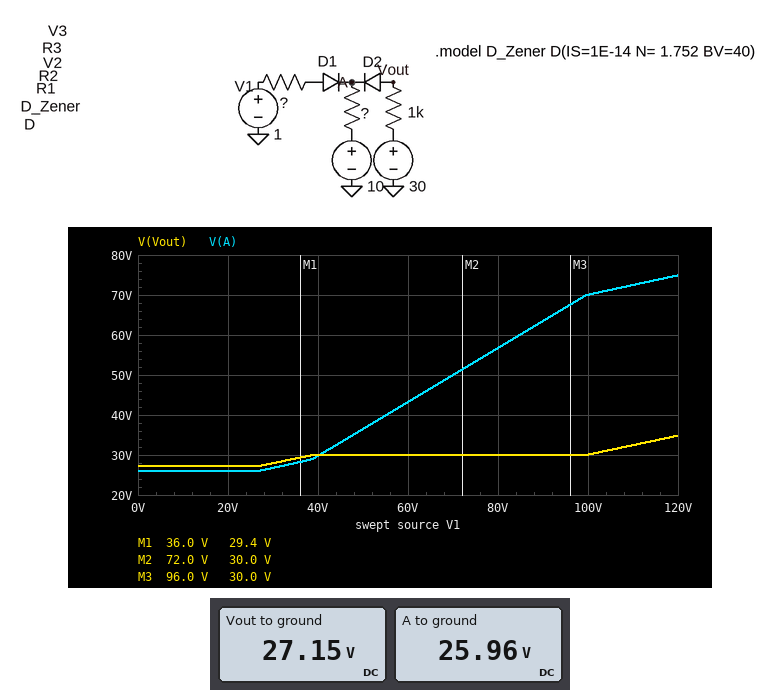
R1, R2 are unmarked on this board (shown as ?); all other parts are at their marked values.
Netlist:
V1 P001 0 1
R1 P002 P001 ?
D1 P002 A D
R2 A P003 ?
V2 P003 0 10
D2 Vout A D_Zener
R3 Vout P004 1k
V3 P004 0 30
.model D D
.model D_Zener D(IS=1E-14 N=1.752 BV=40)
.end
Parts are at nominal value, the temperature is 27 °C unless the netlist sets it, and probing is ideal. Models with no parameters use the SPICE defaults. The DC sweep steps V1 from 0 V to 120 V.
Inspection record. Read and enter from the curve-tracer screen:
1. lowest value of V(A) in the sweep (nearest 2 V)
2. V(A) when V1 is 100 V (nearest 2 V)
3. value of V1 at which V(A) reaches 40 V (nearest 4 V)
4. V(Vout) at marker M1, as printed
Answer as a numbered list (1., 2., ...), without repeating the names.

1. 26 V
2. 70 V
3. 56 V
4. 29.4 V
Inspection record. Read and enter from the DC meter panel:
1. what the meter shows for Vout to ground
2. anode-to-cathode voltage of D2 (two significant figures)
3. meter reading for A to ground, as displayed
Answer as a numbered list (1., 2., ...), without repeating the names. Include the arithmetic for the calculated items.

1. 27.15 V
2. 27.15 V - 25.96 V = 1.2 V
3. 25.96 V
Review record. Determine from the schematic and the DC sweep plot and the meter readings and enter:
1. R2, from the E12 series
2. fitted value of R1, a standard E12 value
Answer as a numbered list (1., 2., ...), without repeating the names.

1. 5.6 kΩ
2. 2.7 kΩ
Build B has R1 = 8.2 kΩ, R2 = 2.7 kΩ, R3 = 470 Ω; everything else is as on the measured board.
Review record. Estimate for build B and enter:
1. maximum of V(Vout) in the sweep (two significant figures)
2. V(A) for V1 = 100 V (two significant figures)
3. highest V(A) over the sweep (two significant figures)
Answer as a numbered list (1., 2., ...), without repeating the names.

1. 30 V
2. 32 V
3. 37 V
